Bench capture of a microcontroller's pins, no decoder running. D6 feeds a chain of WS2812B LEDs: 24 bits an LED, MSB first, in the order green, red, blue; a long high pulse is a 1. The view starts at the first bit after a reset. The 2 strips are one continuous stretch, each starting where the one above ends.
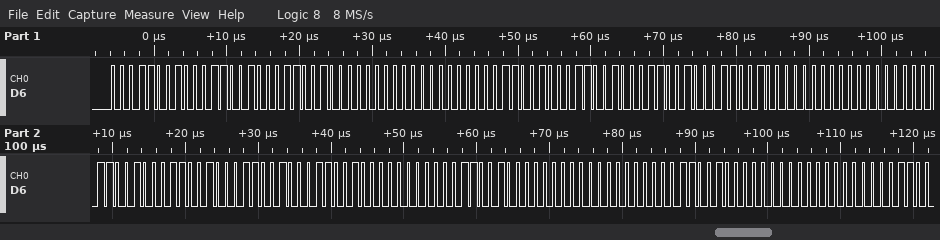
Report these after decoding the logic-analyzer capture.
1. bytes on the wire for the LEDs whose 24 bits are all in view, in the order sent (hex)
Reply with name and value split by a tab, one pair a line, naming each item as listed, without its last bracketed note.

bytes on the wire for the LEDs whose 24 bits are all in view, in the order sent	19 19 19 00 00 19 19 19 19 00 00 19 19 19 19 00 19 00 00 19 00
